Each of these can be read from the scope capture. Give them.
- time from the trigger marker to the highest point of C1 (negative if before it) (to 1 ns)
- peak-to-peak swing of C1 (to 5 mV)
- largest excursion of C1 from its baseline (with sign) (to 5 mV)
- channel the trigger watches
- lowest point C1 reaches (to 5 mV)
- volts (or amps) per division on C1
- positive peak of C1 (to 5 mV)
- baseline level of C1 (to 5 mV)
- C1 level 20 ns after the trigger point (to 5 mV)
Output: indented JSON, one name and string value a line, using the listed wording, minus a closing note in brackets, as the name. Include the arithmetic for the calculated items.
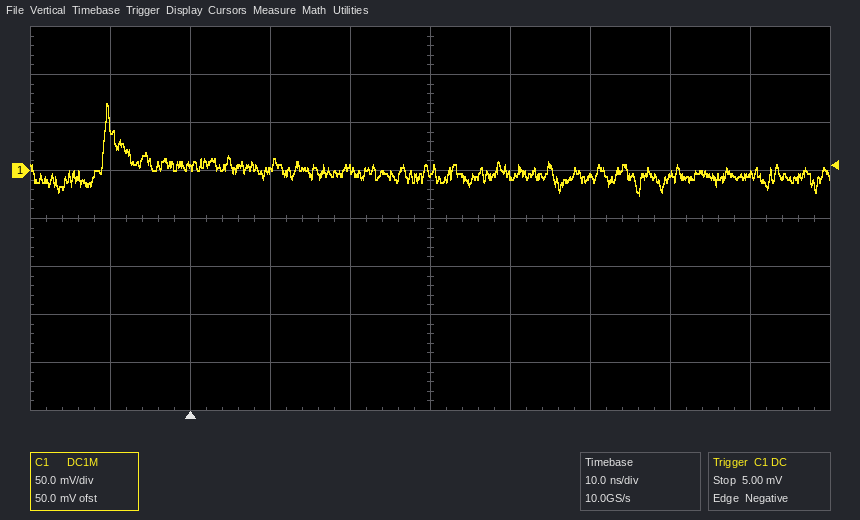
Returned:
{
  "time from the trigger marker to the highest point of C1 (negative if before it)": "-10 ns",
  "peak-to-peak swing of C1": "70 mV − (-25 mV) = 95 mV",
  "largest excursion of C1 from its baseline (with sign)": "70 mV − (-5 mV) = +75 mV",
  "channel the trigger watches": "C1",
  "lowest point C1 reaches": "-25 mV",
  "volts (or amps) per division on C1": "50 mV",
  "positive peak of C1": "70 mV",
  "baseline level of C1": "-5 mV",
  "C1 level 20 ns after the trigger point": "0 mV"
}
